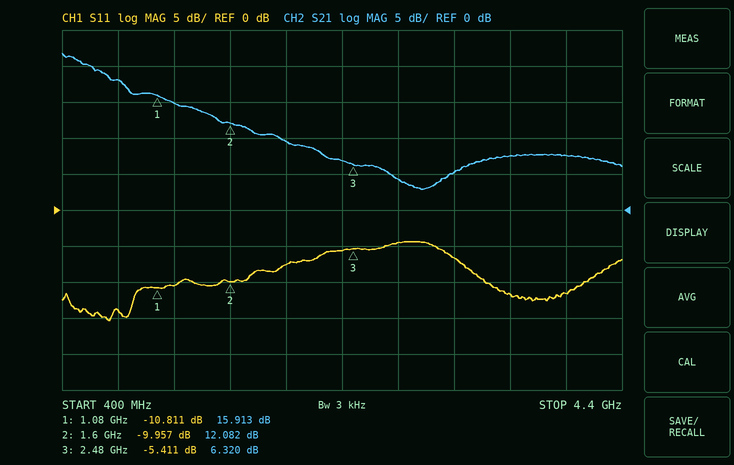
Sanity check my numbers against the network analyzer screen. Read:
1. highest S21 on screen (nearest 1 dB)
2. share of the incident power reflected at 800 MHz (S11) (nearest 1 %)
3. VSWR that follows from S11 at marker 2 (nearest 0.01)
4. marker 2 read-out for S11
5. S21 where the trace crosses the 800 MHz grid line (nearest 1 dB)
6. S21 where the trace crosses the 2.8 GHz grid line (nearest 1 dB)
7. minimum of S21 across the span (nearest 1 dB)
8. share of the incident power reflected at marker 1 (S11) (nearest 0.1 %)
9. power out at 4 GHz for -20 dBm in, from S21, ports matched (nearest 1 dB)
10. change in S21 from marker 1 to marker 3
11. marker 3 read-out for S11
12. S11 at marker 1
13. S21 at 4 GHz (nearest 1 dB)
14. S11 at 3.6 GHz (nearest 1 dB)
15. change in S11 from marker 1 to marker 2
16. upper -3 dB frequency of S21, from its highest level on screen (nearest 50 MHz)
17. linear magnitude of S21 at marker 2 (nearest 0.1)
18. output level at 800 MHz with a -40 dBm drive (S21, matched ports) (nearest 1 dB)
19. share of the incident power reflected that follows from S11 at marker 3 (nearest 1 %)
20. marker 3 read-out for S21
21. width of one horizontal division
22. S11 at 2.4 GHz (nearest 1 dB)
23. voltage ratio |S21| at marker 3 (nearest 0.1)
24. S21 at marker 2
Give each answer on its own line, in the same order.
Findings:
22 dB
4 %
1.93
-9.957 dB
18 dB
4 dB
3 dB
8.3 %
-12 dBm
-9.593 dB
-5.411 dB
-10.811 dB
8 dB
-12 dB
0.854 dB
700 MHz
4.0
-22 dBm
29 %
6.320 dB
400 MHz
-6 dB
2.1
12.082 dB
